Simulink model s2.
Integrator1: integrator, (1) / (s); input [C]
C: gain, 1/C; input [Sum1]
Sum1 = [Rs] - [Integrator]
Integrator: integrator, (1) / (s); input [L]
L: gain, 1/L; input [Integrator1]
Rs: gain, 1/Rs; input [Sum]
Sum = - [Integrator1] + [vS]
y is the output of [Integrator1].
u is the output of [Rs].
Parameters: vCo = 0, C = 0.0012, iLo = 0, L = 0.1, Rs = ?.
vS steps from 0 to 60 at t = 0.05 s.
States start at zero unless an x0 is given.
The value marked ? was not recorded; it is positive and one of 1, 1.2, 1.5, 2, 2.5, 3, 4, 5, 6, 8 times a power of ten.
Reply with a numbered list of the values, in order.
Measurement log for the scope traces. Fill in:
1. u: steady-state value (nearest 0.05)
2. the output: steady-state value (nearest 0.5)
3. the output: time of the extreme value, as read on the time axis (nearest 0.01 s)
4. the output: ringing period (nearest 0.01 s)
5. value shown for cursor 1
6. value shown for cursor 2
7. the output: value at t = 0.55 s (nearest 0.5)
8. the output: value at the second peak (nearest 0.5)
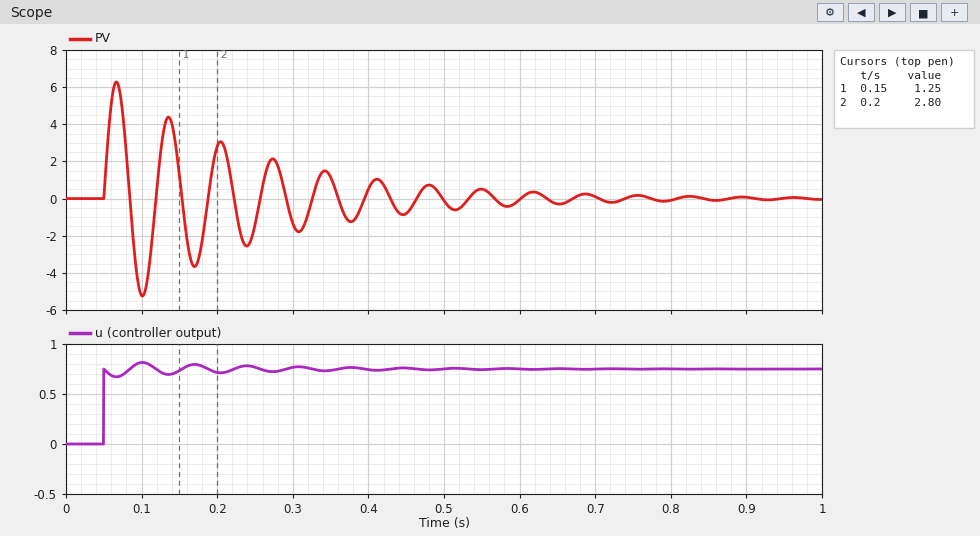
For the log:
1. 0.75
2. 0.0
3. 0.07 s
4. 0.07 s
5. 1.25
6. 2.80
7. 0.5
8. 4.5
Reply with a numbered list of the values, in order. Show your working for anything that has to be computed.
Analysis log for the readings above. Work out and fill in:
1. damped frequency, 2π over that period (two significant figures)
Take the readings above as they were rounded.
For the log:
1. 2π / 0.07 = 90 rad/s
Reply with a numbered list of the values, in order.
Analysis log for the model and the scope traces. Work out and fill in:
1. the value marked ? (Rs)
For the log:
1. 80
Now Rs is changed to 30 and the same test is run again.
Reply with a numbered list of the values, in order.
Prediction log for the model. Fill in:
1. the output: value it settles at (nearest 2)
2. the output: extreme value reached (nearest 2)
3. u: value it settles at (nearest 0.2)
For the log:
1. 0
2. 14
3. 2.0
